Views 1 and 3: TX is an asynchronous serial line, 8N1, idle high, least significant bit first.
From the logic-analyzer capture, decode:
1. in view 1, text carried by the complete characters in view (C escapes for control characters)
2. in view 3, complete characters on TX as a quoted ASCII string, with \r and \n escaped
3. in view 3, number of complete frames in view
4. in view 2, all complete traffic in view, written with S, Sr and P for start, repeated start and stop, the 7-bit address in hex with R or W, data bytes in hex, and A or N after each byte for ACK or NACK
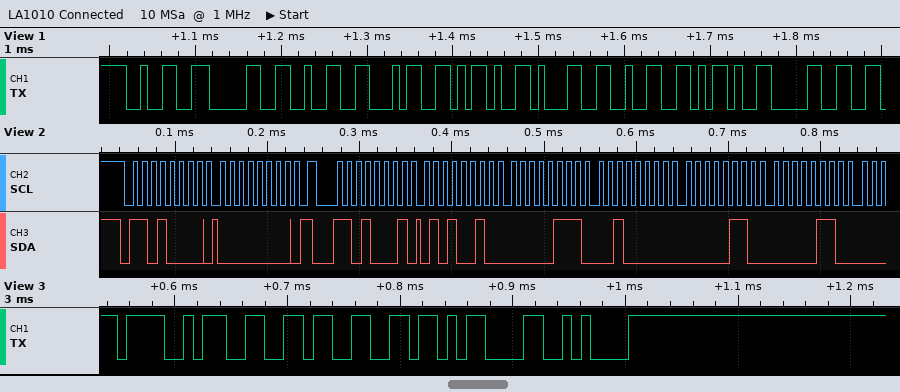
"2024-12-0"
"Off\r\n"
5
S 68W A 00 A Sr 68R A 52 A 07 A 20 A 06 A 06 A
